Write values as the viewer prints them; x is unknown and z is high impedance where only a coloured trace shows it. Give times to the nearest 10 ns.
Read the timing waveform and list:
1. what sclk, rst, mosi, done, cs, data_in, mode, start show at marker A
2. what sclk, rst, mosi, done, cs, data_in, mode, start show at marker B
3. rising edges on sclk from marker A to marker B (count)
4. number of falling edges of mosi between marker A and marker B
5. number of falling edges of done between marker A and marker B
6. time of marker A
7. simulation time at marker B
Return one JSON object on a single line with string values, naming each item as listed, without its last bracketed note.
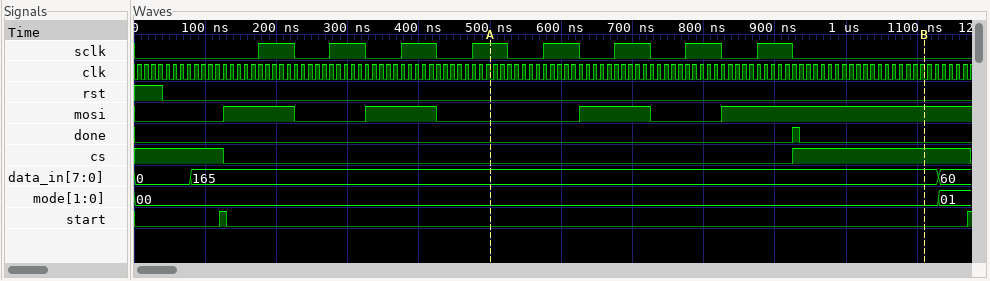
{"what sclk, rst, mosi, done, cs, data_in, mode, start show at marker A": "sclk=1, rst=0, mosi=0, done=0, cs=0, data_in=165, mode=00, start=0", "what sclk, rst, mosi, done, cs, data_in, mode, start show at marker B": "sclk=0, rst=0, mosi=1, done=0, cs=1, data_in=165, mode=00, start=0", "rising edges on sclk from marker A to marker B": "4", "number of falling edges of mosi between marker A and marker B": "1", "number of falling edges of done between marker A and marker B": "1", "time of marker A": "500 ns", "simulation time at marker B": "1110 ns"}
